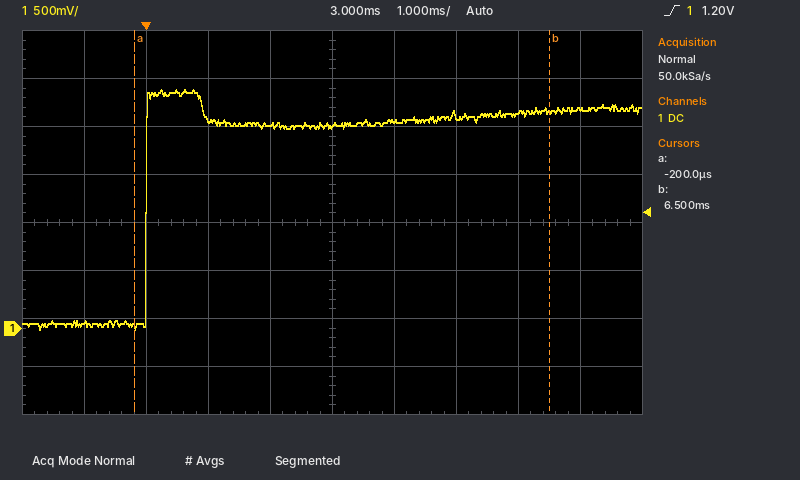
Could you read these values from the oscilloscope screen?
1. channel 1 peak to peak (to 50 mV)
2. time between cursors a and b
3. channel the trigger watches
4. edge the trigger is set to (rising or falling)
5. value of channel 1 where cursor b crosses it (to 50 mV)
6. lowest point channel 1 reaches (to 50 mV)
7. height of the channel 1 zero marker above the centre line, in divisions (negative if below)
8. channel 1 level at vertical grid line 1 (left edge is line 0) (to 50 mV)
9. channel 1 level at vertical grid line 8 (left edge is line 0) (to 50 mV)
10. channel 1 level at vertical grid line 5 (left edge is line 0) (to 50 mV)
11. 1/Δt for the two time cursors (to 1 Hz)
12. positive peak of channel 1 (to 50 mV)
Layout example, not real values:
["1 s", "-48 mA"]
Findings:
["2.50 V", "6.7 ms", "channel 1", "rising", "2.25 V", "0 mV", "-2.2 div", "50 mV", "2.25 V", "2.10 V", "149 Hz", "2.50 V"]
